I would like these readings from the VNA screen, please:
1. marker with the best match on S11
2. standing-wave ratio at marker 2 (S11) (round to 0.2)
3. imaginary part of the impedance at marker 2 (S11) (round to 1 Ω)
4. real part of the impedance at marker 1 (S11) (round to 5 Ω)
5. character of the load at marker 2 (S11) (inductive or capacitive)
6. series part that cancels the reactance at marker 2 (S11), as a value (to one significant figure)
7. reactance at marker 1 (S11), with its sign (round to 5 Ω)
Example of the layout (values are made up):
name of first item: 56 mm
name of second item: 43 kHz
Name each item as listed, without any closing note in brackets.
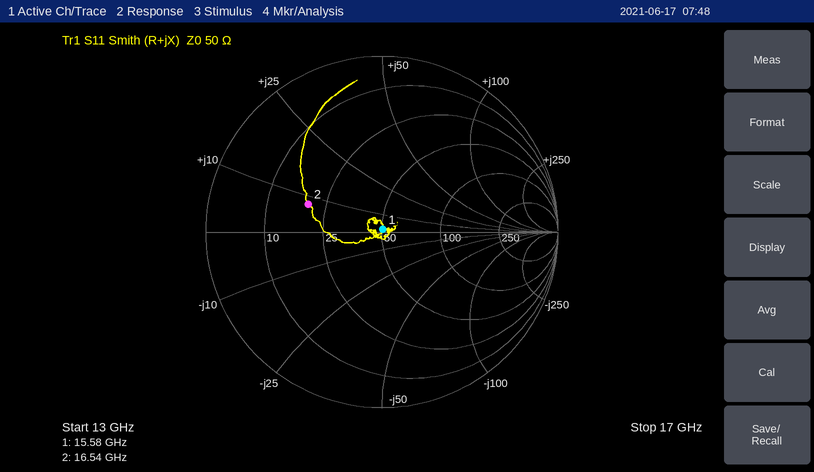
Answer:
marker with the best match on S11: marker 1
standing-wave ratio at marker 2 (S11): 2.6
imaginary part of the impedance at marker 2 (S11): +8 Ω
real part of the impedance at marker 1 (S11): 50 Ω
character of the load at marker 2 (S11): inductive
series part that cancels the reactance at marker 2 (S11), as a value: 1 pF
reactance at marker 1 (S11), with its sign: 0 Ω
